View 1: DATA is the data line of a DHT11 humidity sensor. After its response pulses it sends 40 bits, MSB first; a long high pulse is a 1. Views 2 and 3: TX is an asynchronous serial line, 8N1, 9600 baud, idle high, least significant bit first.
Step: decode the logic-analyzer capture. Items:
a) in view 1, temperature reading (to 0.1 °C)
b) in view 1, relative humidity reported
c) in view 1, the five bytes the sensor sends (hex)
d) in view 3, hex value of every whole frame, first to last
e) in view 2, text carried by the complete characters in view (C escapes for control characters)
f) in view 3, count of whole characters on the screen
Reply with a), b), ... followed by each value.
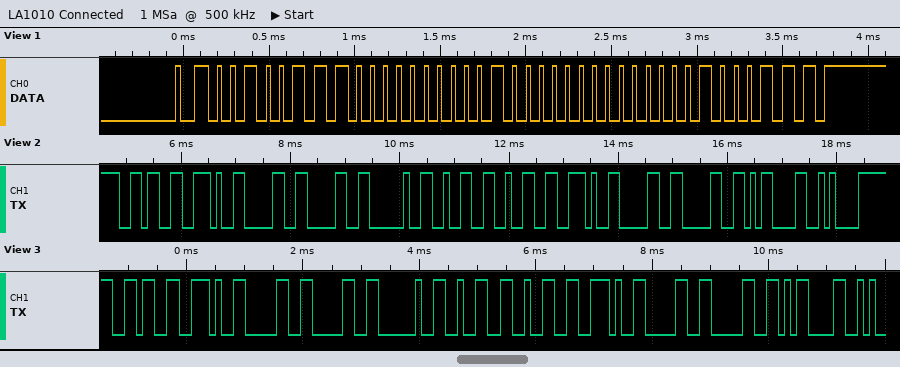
a) 32.0 °C
b) 39 %
c) 27 00 20 00 47
d) 0x36 0x2E 0x30 0x30 0x20 0x32 0x32 0x2E 0x30 0x30 0x0D
e) "6.00 22.00\r\n"
f) 11
